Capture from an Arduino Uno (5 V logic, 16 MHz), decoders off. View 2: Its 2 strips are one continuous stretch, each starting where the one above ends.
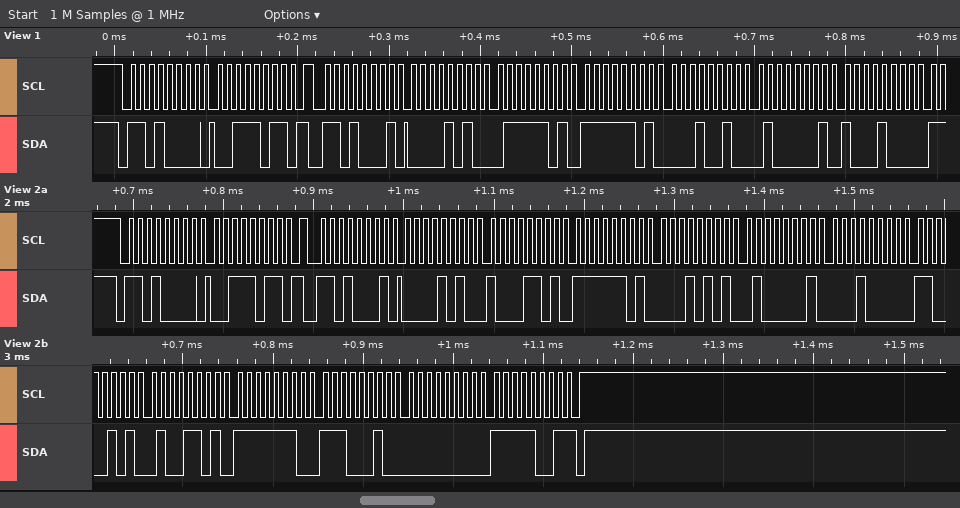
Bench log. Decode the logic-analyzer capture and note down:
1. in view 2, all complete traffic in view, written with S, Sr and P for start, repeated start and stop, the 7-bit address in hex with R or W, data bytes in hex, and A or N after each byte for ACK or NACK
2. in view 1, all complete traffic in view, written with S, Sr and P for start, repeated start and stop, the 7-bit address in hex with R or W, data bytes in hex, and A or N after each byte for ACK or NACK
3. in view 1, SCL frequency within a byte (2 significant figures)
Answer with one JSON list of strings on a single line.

["S 68W A 3B A Sr 68R A 0A A 8D A FD A 15 A 41 A 10 A C5 A 4D A FE A E2 A 00 A F9 N P", "S 68W A 3B A Sr 68R A 0A A 7D A FD A 12 A 41 A 88 A", "100 kHz"]
